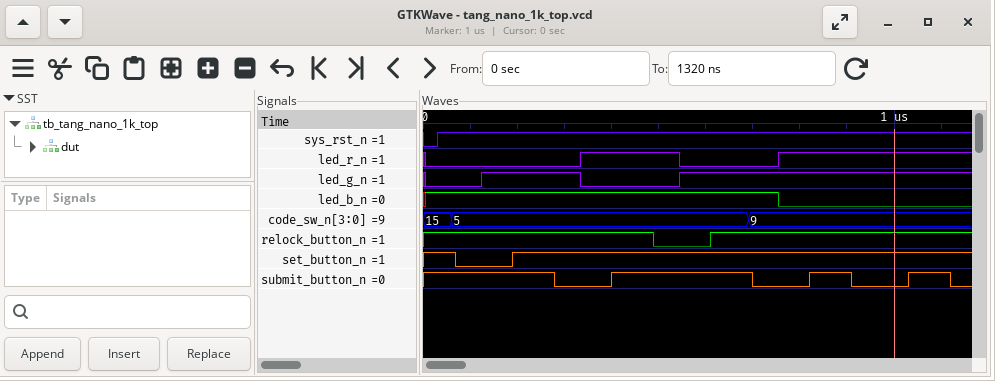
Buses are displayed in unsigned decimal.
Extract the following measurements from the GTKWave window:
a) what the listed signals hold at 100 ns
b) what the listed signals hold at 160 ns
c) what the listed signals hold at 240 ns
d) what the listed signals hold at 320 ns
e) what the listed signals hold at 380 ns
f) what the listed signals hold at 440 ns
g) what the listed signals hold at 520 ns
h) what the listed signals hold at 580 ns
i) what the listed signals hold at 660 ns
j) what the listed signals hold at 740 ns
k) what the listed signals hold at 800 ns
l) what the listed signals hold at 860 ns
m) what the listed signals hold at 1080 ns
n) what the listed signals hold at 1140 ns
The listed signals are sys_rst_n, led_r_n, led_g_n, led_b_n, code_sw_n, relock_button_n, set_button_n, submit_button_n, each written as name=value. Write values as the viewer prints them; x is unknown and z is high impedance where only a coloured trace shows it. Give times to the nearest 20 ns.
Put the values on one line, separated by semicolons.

sys_rst_n=1, led_r_n=0, led_g_n=0, led_b_n=1, code_sw_n=5, relock_button_n=1, set_button_n=0, submit_button_n=1; sys_rst_n=1, led_r_n=0, led_g_n=1, led_b_n=1, code_sw_n=5, relock_button_n=1, set_button_n=0, submit_button_n=1; sys_rst_n=1, led_r_n=0, led_g_n=1, led_b_n=1, code_sw_n=5, relock_button_n=1, set_button_n=1, submit_button_n=1; sys_rst_n=1, led_r_n=0, led_g_n=1, led_b_n=1, code_sw_n=5, relock_button_n=1, set_button_n=1, submit_button_n=0; sys_rst_n=1, led_r_n=1, led_g_n=0, led_b_n=1, code_sw_n=5, relock_button_n=1, set_button_n=1, submit_button_n=0; sys_rst_n=1, led_r_n=1, led_g_n=0, led_b_n=1, code_sw_n=5, relock_button_n=1, set_button_n=1, submit_button_n=1; sys_rst_n=1, led_r_n=1, led_g_n=0, led_b_n=1, code_sw_n=5, relock_button_n=0, set_button_n=1, submit_button_n=1; sys_rst_n=1, led_r_n=0, led_g_n=1, led_b_n=1, code_sw_n=5, relock_button_n=0, set_button_n=1, submit_button_n=1; sys_rst_n=1, led_r_n=0, led_g_n=1, led_b_n=1, code_sw_n=5, relock_button_n=1, set_button_n=1, submit_button_n=1; sys_rst_n=1, led_r_n=0, led_g_n=1, led_b_n=1, code_sw_n=9, relock_button_n=1, set_button_n=1, submit_button_n=0; sys_rst_n=1, led_r_n=1, led_g_n=1, led_b_n=0, code_sw_n=9, relock_button_n=1, set_button_n=1, submit_button_n=0; sys_rst_n=1, led_r_n=1, led_g_n=1, led_b_n=0, code_sw_n=9, relock_button_n=1, set_button_n=1, submit_button_n=1; sys_rst_n=1, led_r_n=1, led_g_n=1, led_b_n=0, code_sw_n=9, relock_button_n=1, set_button_n=1, submit_button_n=1; sys_rst_n=1, led_r_n=1, led_g_n=1, led_b_n=0, code_sw_n=9, relock_button_n=1, set_button_n=1, submit_button_n=0
